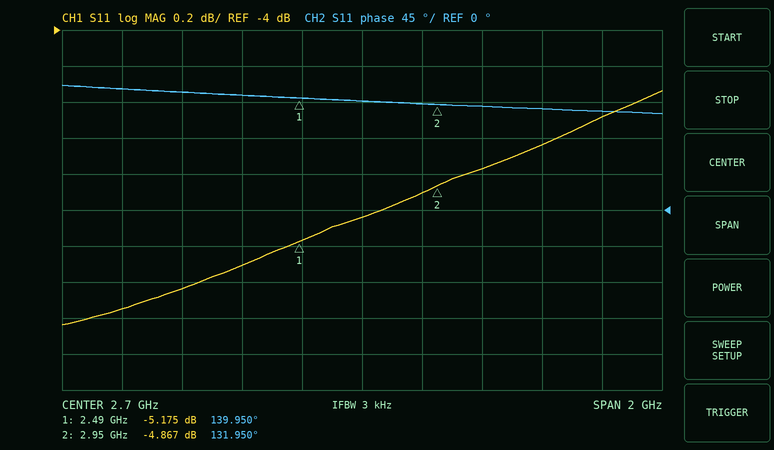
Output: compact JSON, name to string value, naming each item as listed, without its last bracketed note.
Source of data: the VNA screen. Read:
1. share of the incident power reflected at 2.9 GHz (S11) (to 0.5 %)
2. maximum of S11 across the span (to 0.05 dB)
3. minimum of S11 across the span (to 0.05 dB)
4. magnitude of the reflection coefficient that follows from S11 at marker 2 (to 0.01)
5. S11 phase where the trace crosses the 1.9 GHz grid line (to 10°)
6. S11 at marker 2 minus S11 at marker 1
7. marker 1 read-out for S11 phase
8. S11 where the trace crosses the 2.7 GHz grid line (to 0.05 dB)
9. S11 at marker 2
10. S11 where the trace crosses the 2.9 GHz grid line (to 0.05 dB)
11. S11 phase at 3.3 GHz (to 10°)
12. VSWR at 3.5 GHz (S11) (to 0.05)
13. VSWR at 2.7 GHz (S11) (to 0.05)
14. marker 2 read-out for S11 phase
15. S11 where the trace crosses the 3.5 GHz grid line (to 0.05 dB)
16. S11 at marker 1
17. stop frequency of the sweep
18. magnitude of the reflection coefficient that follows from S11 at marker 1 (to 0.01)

{"share of the incident power reflected at 2.9 GHz (S11)": "32.5 %", "maximum of S11 across the span": "-4.35 dB", "minimum of S11 across the span": "-5.65 dB", "magnitude of the reflection coefficient that follows from S11 at marker 2": "0.57", "S11 phase where the trace crosses the 1.9 GHz grid line": "150°", "S11 at marker 2 minus S11 at marker 1": "0.308 dB", "marker 1 read-out for S11 phase": "139.950°", "S11 where the trace crosses the 2.7 GHz grid line": "-5.05 dB", "S11 at marker 2": "-4.867 dB", "S11 where the trace crosses the 2.9 GHz grid line": "-4.90 dB", "S11 phase at 3.3 GHz": "130°", "VSWR at 3.5 GHz (S11)": "3.95", "VSWR at 2.7 GHz (S11)": "3.55", "marker 2 read-out for S11 phase": "131.950°", "S11 where the trace crosses the 3.5 GHz grid line": "-4.50 dB", "S11 at marker 1": "-5.175 dB", "stop frequency of the sweep": "3.7 GHz", "magnitude of the reflection coefficient that follows from S11 at marker 1": "0.55"}
